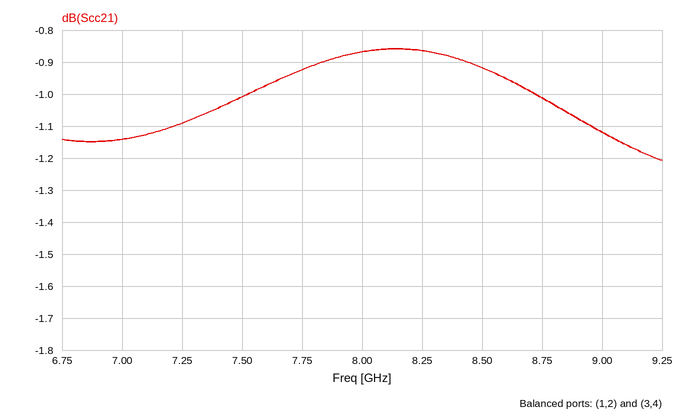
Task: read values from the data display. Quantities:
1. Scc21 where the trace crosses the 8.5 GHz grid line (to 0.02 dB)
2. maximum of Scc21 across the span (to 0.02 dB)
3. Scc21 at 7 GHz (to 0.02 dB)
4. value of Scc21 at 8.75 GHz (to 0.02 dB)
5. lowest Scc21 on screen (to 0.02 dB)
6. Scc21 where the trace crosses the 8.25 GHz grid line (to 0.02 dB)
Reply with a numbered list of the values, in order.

1. -0.92 dB
2. -0.86 dB
3. -1.14 dB
4. -1.02 dB
5. -1.20 dB
6. -0.86 dB
